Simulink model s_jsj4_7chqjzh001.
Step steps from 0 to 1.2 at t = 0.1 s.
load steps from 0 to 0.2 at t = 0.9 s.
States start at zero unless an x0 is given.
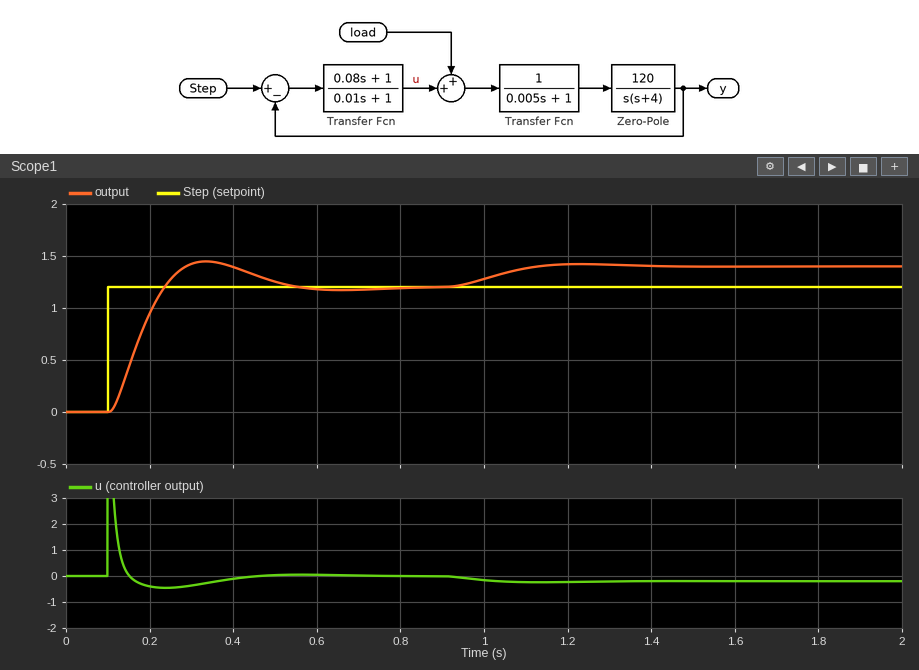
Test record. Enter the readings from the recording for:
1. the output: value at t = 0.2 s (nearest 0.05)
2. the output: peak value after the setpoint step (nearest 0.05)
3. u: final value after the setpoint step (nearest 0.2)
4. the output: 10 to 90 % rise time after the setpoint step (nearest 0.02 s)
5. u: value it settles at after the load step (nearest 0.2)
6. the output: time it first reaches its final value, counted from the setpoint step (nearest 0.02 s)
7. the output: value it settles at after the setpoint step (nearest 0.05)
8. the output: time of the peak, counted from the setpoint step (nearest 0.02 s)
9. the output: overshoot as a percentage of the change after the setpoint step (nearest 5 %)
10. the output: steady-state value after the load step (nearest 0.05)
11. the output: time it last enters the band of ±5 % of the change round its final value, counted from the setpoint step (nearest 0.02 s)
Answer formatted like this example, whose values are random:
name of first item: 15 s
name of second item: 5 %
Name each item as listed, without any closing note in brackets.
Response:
the output: value at t = 0.2 s: 0.95
the output: peak value after the setpoint step: 1.45
u: final value after the setpoint step: 0.0
the output: 10 to 90 % rise time after the setpoint step: 0.10 s
u: value it settles at after the load step: -0.2
the output: time it first reaches its final value, counted from the setpoint step: 0.14 s
the output: value it settles at after the setpoint step: 1.20
the output: time of the peak, counted from the setpoint step: 0.24 s
the output: overshoot as a percentage of the change after the setpoint step: 20 %
the output: steady-state value after the load step: 1.40
the output: time it last enters the band of ±5 % of the change round its final value, counted from the setpoint step: 0.40 s
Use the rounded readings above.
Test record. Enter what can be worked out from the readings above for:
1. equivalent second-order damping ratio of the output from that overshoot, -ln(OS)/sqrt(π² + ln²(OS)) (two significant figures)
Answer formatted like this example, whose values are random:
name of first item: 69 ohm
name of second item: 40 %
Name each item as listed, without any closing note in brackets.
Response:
equivalent second-order damping ratio of the output from that overshoot, -ln(OS)/sqrt(π² + ln²(OS)): 0.46
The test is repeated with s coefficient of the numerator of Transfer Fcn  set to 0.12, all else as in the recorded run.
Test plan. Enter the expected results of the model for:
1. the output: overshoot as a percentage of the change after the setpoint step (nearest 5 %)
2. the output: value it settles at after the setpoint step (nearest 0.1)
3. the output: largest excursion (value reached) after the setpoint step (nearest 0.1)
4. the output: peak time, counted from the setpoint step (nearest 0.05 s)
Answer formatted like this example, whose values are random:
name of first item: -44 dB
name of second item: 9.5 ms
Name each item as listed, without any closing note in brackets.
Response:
the output: overshoot as a percentage of the change after the setpoint step: 10 %
the output: value it settles at after the setpoint step: 1.2
the output: largest excursion (value reached) after the setpoint step: 1.3
the output: peak time, counted from the setpoint step: 0.20 s
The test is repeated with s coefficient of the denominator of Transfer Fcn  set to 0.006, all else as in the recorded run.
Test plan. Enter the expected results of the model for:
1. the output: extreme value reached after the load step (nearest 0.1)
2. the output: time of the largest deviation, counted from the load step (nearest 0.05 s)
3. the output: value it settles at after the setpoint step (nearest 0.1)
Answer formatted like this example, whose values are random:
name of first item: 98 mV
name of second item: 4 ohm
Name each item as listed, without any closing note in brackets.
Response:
the output: extreme value reached after the load step: 1.4
the output: time of the largest deviation, counted from the load step: 0.35 s
the output: value it settles at after the setpoint step: 1.2
